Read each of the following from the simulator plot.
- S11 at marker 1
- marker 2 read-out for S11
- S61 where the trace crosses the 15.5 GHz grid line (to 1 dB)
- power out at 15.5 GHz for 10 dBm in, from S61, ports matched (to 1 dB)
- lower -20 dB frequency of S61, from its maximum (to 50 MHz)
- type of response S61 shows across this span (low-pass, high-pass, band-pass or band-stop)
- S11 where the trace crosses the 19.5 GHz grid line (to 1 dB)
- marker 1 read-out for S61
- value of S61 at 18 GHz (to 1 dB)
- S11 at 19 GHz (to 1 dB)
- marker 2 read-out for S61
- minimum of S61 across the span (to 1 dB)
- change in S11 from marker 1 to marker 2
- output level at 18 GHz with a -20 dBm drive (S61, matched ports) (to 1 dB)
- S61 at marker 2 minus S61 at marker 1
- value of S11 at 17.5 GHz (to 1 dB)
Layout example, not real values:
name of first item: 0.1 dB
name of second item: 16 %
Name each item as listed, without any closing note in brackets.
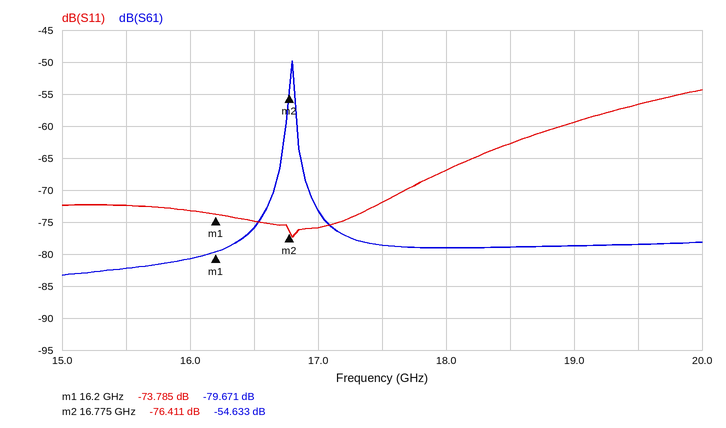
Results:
S11 at marker 1: -73.785 dB
marker 2 read-out for S11: -76.411 dB
S61 where the trace crosses the 15.5 GHz grid line: -82 dB
power out at 15.5 GHz for 10 dBm in, from S61, ports matched: -72 dBm
lower -20 dB frequency of S61, from its maximum: 16.65 GHz
type of response S61 shows across this span: band-pass
S11 where the trace crosses the 19.5 GHz grid line: -57 dB
marker 1 read-out for S61: -79.671 dB
value of S61 at 18 GHz: -79 dB
S11 at 19 GHz: -59 dB
marker 2 read-out for S61: -54.633 dB
minimum of S61 across the span: -83 dB
change in S11 from marker 1 to marker 2: -2.626 dB
output level at 18 GHz with a -20 dBm drive (S61, matched ports): -99 dBm
S61 at marker 2 minus S61 at marker 1: 25.038 dB
value of S11 at 17.5 GHz: -72 dB
